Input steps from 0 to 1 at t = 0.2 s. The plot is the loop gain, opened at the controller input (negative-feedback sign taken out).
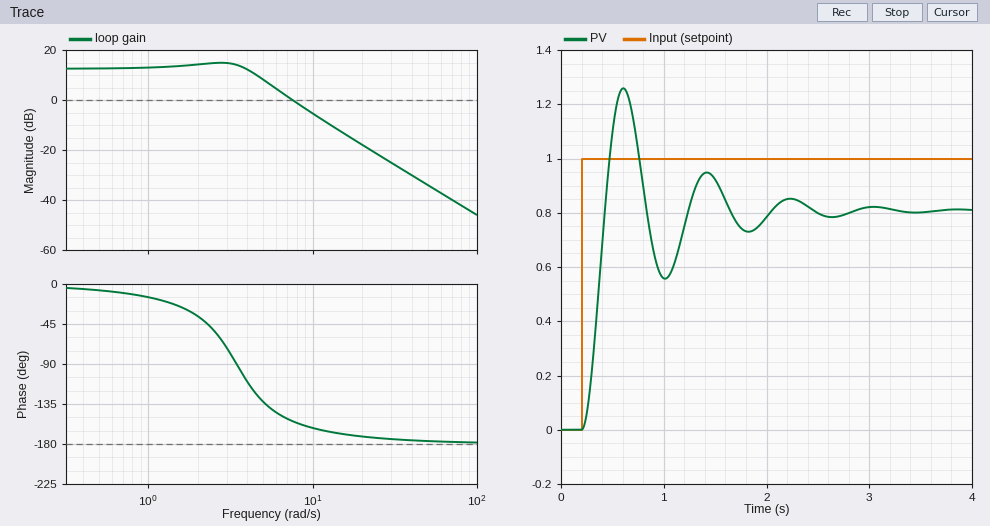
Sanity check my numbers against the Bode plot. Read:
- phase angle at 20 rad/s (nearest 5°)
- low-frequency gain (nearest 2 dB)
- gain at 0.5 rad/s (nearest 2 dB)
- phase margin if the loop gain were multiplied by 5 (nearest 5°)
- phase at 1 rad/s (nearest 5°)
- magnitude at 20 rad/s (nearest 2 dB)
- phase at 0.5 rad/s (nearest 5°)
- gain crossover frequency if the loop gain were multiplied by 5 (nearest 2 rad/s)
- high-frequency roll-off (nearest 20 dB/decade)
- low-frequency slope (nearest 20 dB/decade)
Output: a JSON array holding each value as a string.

["-170°", "12 dB", "12 dB", "10°", "-15°", "-18 dB", "-5°", "16 rad/s", "-40 dB/decade", "0 dB/decade"]
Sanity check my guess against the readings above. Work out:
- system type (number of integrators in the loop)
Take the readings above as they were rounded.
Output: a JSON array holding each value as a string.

["0"]
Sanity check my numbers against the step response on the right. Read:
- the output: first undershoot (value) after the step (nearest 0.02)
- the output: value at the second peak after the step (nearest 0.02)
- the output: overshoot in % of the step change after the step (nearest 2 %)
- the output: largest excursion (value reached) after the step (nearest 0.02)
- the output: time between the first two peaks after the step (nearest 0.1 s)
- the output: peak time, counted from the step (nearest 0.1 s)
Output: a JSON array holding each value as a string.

["0.56", "0.94", "56 %", "1.26", "0.8 s", "0.4 s"]
